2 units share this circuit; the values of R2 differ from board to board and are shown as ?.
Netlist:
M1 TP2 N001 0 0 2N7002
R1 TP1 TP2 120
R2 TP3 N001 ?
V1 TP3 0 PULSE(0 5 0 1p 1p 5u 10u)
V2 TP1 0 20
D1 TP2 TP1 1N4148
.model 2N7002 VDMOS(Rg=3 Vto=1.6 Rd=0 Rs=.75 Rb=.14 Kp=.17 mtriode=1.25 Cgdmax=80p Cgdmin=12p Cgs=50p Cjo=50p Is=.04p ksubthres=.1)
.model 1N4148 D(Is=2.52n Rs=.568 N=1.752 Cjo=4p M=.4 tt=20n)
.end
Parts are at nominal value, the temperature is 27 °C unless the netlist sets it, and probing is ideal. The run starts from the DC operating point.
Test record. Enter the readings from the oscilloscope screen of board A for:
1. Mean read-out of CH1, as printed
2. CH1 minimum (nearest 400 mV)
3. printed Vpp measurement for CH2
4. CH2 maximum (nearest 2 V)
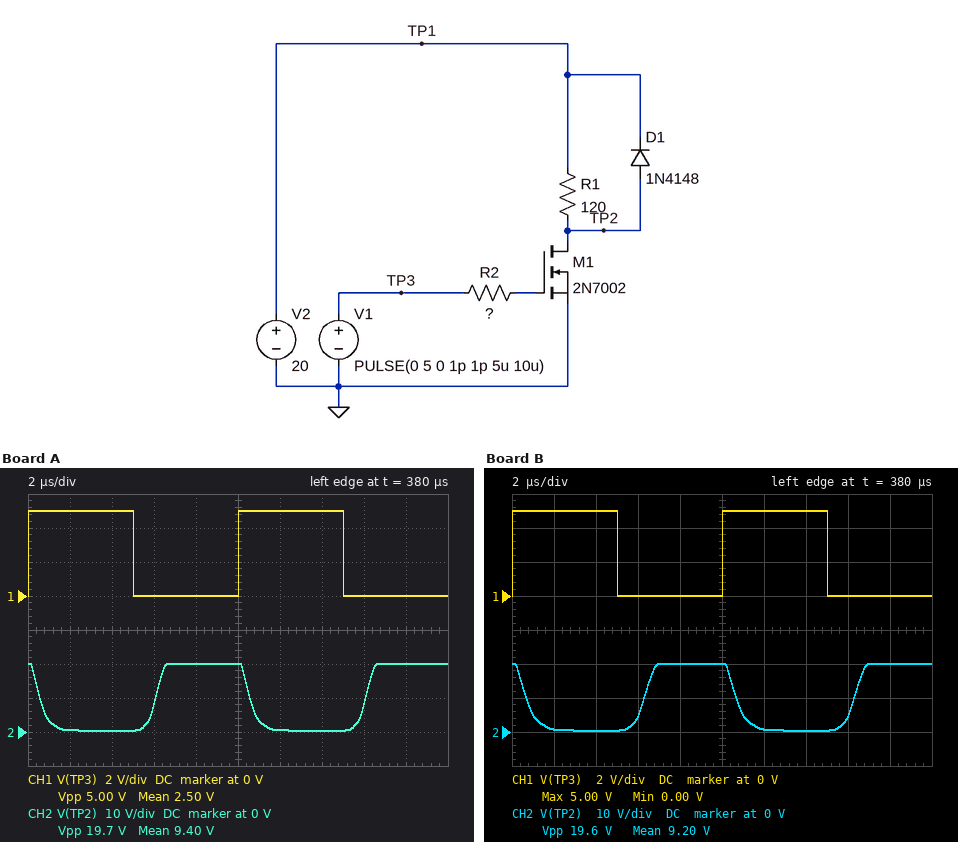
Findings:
2.50 V
0 V
19.7 V
20 V
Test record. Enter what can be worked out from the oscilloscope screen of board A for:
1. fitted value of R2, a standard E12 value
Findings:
5.6 kΩ
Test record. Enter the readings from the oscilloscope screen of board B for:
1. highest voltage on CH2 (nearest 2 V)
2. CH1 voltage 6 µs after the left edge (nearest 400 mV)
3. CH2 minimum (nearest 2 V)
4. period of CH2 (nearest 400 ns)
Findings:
20 V
0 V
0 V
10.0 µs
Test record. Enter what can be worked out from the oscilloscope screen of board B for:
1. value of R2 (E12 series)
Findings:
6.8 kΩ
